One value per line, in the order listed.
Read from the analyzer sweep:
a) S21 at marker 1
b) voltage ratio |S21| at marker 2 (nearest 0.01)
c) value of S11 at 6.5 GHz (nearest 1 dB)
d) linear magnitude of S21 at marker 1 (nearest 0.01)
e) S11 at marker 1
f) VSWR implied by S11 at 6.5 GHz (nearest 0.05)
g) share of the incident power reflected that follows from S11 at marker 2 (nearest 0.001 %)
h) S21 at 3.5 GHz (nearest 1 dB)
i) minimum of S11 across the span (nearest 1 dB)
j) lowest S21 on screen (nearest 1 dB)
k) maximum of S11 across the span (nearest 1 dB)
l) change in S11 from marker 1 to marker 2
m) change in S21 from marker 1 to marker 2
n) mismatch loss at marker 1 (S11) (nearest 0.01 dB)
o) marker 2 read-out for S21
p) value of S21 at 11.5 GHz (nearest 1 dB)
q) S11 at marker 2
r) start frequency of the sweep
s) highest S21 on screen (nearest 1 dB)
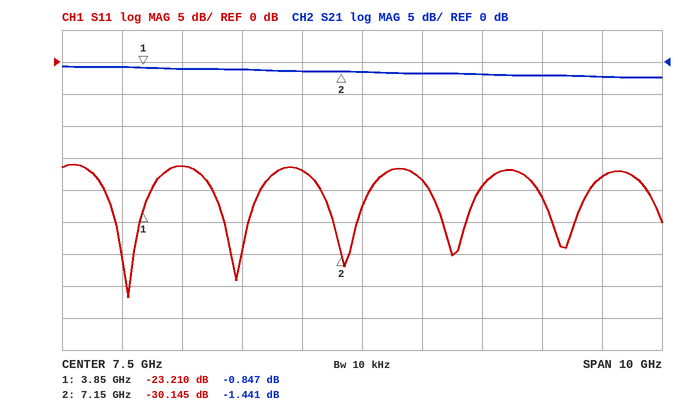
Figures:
-0.847 dB
0.85
-17 dB
0.91
-23.210 dB
1.35
0.097 %
-1 dB
-37 dB
-2 dB
-16 dB
-6.935 dB
-0.594 dB
0.02 dB
-1.441 dB
-2 dB
-30.145 dB
2.5 GHz
-1 dB
